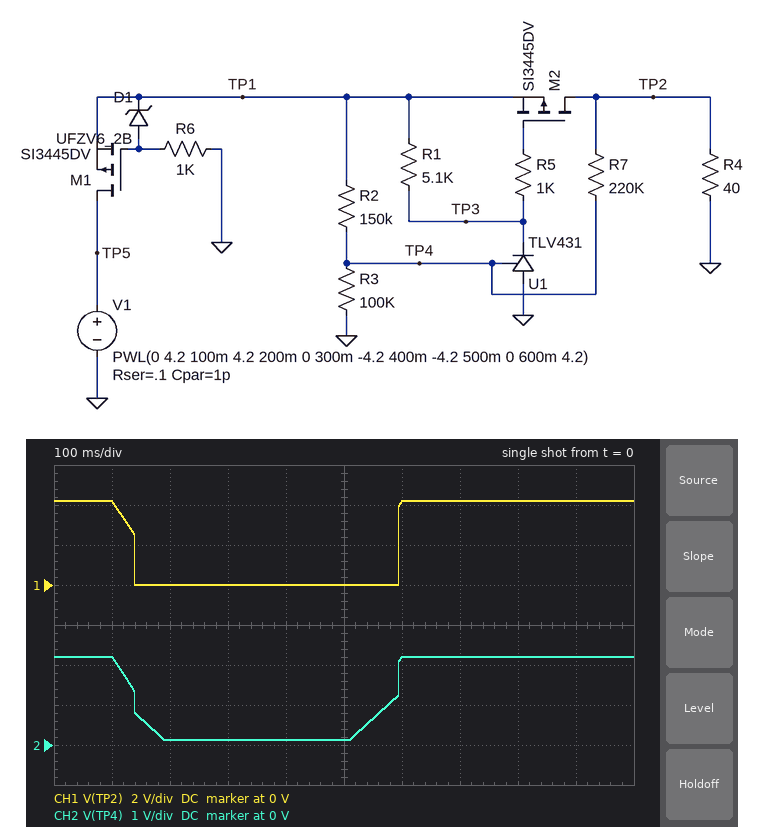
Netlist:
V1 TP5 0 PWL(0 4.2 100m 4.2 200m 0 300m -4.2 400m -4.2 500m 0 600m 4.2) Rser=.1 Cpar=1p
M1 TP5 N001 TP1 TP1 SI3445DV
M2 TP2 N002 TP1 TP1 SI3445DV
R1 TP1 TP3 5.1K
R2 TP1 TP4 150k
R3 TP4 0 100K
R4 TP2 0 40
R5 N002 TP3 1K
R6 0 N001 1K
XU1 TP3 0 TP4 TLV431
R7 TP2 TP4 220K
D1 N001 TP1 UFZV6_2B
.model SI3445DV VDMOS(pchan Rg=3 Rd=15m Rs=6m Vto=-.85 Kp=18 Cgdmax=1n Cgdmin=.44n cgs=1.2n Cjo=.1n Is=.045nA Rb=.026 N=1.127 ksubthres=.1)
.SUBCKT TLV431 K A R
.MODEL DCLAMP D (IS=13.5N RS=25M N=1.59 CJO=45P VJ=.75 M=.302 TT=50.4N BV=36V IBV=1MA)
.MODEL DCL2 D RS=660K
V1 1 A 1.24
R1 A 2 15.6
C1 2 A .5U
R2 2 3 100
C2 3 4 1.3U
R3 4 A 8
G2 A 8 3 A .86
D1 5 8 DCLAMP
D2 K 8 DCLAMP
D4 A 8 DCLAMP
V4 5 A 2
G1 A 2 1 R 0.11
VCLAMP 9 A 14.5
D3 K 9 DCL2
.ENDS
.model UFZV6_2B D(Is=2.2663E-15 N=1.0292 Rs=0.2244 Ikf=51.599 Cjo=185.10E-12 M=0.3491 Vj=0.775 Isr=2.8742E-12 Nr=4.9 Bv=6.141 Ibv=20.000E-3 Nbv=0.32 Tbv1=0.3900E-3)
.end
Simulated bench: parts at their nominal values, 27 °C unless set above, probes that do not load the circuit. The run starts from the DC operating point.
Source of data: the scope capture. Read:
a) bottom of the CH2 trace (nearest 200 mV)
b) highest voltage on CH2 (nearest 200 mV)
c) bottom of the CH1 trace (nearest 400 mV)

200 mV
2.2 V
0 V
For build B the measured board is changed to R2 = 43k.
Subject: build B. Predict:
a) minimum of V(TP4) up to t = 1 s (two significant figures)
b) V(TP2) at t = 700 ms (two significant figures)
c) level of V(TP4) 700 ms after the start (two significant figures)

250 mV
4.2 V
3.1 V
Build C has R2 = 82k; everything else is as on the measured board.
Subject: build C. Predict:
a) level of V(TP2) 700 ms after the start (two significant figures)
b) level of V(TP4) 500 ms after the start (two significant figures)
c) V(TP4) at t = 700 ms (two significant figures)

4.2 V
190 mV
2.6 V
